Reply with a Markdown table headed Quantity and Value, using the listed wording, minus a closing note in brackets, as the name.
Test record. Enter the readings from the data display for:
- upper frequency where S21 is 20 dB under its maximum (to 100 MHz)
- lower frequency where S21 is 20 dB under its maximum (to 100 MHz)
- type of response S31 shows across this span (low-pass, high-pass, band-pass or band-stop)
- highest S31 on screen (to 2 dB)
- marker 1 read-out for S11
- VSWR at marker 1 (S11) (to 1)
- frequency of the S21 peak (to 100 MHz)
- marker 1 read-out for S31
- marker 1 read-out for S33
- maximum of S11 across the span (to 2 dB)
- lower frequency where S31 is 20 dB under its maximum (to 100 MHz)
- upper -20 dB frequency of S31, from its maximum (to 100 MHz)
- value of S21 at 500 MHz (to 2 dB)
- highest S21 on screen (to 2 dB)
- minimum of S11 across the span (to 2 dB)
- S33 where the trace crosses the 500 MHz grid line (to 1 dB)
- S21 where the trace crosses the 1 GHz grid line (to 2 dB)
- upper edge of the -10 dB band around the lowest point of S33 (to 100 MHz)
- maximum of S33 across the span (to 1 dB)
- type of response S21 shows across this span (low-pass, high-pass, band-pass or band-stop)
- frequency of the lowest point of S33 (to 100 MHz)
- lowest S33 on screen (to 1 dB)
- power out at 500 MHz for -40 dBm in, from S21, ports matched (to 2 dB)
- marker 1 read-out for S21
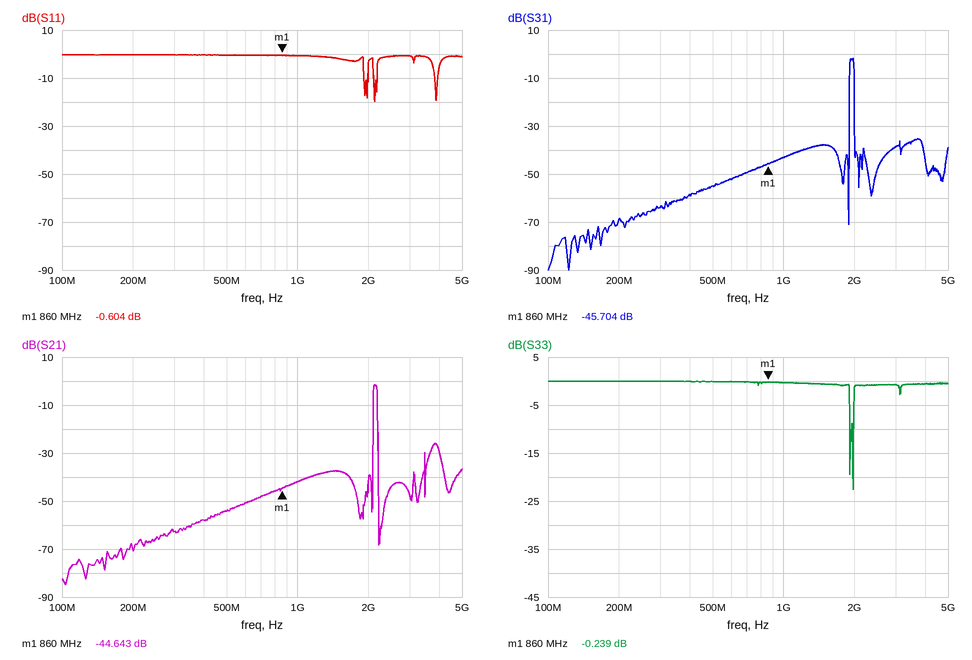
| Quantity | Value |
|---|---|
| upper frequency where S21 is 20 dB under its maximum | 2.2 GHz |
| lower frequency where S21 is 20 dB under its maximum | 2.1 GHz |
| type of response S31 shows across this span | band-pass |
| highest S31 on screen | -2 dB |
| marker 1 read-out for S11 | -0.604 dB |
| VSWR at marker 1 (S11) | 29 |
| frequency of the S21 peak | 2.1 GHz |
| marker 1 read-out for S31 | -45.704 dB |
| marker 1 read-out for S33 | -0.239 dB |
| maximum of S11 across the span | 0 dB |
| lower frequency where S31 is 20 dB under its maximum | 1.9 GHz |
| upper -20 dB frequency of S31, from its maximum | 2.0 GHz |
| value of S21 at 500 MHz | -54 dB |
| highest S21 on screen | -2 dB |
| minimum of S11 across the span | -20 dB |
| S33 where the trace crosses the 500 MHz grid line | 0 dB |
| S21 where the trace crosses the 1 GHz grid line | -42 dB |
| upper edge of the -10 dB band around the lowest point of S33 | 2.0 GHz |
| maximum of S33 across the span | 0 dB |
| type of response S21 shows across this span | band-pass |
| frequency of the lowest point of S33 | 2.0 GHz |
| lowest S33 on screen | -23 dB |
| power out at 500 MHz for -40 dBm in, from S21, ports matched | -94 dBm |
| marker 1 read-out for S21 | -44.643 dB |
